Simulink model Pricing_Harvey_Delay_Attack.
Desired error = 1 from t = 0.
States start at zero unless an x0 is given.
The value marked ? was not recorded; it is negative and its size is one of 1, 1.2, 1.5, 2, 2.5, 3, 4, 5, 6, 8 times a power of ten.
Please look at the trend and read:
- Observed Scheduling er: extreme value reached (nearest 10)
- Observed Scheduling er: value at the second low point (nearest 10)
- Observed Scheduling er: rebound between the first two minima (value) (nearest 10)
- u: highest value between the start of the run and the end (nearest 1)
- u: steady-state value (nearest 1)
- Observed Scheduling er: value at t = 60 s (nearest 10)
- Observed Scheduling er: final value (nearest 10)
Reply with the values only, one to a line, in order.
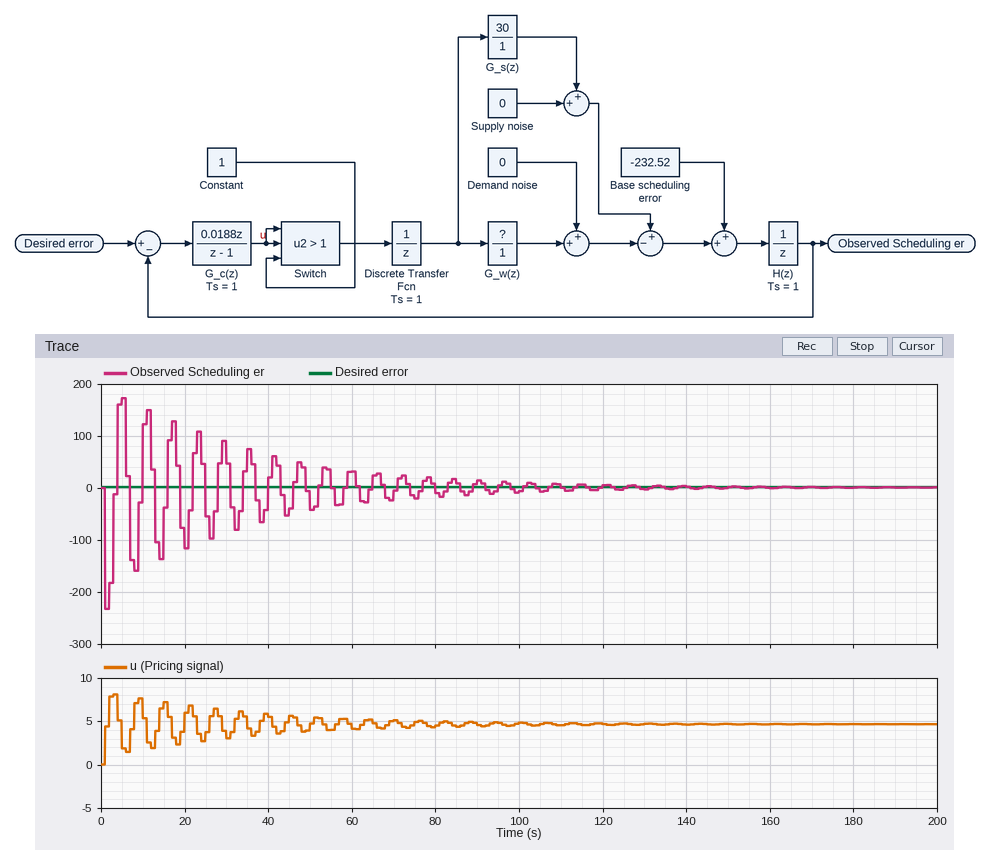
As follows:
-230
-160
170
8
5
30
0
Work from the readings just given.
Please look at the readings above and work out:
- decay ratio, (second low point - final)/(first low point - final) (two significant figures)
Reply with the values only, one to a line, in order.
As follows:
0.70
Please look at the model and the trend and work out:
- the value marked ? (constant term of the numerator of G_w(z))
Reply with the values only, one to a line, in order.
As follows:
-20
